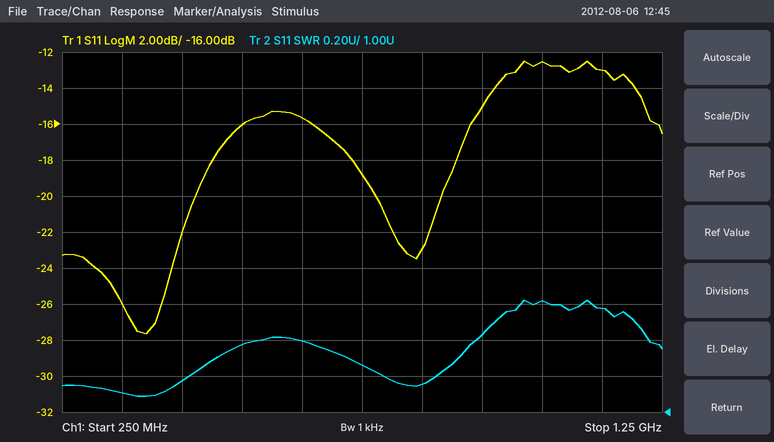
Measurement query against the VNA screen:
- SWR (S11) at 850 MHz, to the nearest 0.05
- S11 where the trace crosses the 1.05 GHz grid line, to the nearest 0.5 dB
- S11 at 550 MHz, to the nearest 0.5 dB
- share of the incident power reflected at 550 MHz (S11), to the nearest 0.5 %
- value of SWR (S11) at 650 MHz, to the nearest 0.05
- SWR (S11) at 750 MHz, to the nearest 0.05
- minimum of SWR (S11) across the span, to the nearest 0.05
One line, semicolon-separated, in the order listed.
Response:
1.15; -12.5 dB; -16.0 dB; 2.5 %; 1.40; 1.25; 1.10
